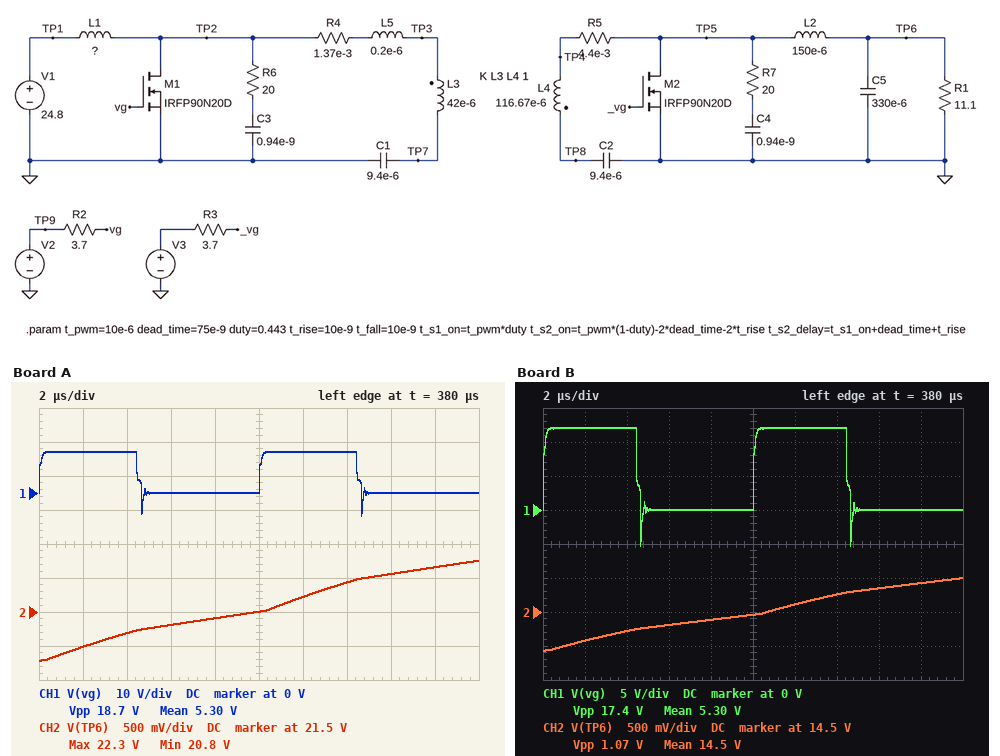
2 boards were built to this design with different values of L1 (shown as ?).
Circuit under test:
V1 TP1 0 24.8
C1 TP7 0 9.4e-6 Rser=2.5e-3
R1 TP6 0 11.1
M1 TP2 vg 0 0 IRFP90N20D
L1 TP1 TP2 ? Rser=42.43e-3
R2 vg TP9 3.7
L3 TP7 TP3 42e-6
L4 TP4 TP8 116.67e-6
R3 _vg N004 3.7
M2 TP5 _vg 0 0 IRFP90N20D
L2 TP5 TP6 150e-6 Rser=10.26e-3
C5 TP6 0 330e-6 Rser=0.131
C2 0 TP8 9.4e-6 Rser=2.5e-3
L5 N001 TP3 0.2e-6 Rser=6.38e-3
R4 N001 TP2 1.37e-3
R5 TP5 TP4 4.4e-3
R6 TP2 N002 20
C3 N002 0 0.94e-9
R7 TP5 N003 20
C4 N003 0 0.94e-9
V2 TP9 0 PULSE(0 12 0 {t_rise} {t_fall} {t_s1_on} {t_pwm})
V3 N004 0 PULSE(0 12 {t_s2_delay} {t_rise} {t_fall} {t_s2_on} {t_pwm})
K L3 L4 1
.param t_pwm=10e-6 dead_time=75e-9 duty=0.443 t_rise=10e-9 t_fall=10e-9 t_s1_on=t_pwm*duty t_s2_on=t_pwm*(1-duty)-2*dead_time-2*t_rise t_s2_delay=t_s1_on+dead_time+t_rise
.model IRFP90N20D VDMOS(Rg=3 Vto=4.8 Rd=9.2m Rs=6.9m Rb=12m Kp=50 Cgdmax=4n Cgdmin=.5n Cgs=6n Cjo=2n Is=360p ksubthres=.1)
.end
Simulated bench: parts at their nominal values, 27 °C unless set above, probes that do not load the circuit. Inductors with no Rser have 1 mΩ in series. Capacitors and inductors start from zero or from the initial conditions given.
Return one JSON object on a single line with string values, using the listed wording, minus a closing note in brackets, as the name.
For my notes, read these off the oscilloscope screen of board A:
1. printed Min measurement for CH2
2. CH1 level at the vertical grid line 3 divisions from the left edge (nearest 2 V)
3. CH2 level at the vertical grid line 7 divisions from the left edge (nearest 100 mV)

{"printed Min measurement for CH2": "20.8 V", "CH1 level at the vertical grid line 3 divisions from the left edge": "0 V", "CH2 level at the vertical grid line 7 divisions from the left edge": "21.9 V"}
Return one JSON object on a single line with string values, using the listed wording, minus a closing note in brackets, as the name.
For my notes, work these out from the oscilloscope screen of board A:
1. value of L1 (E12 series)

{"value of L1": "68 µH"}
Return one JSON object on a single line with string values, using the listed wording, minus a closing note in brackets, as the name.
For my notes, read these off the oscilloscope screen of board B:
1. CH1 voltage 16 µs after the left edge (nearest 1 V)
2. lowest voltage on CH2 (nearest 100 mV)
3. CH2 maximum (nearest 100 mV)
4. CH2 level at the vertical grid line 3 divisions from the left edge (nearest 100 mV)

{"CH1 voltage 16 µs after the left edge": "0 V", "lowest voltage on CH2": "13.9 V", "CH2 maximum": "15.0 V", "CH2 level at the vertical grid line 3 divisions from the left edge": "14.3 V"}
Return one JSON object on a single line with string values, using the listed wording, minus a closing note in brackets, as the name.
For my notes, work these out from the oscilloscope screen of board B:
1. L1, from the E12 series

{"L1, from the E12 series": "180 µH"}
